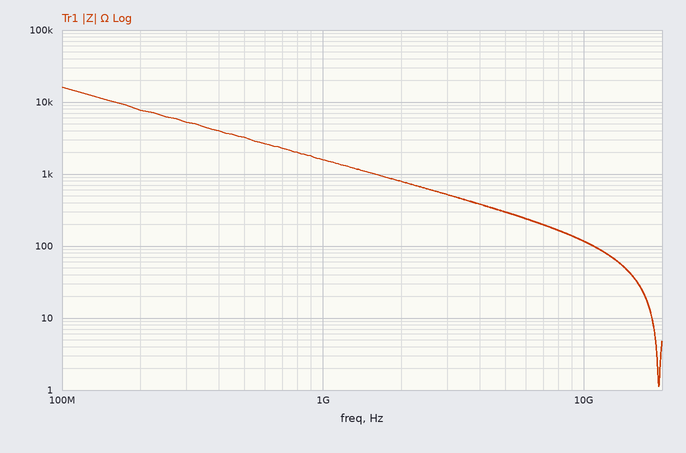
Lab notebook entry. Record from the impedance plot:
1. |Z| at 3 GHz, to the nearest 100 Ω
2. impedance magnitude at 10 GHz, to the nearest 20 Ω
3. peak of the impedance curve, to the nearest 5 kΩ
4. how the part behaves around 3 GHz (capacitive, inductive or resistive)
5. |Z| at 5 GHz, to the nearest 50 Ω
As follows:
500 Ω
120 Ω
15 kΩ
capacitive
300 Ω
